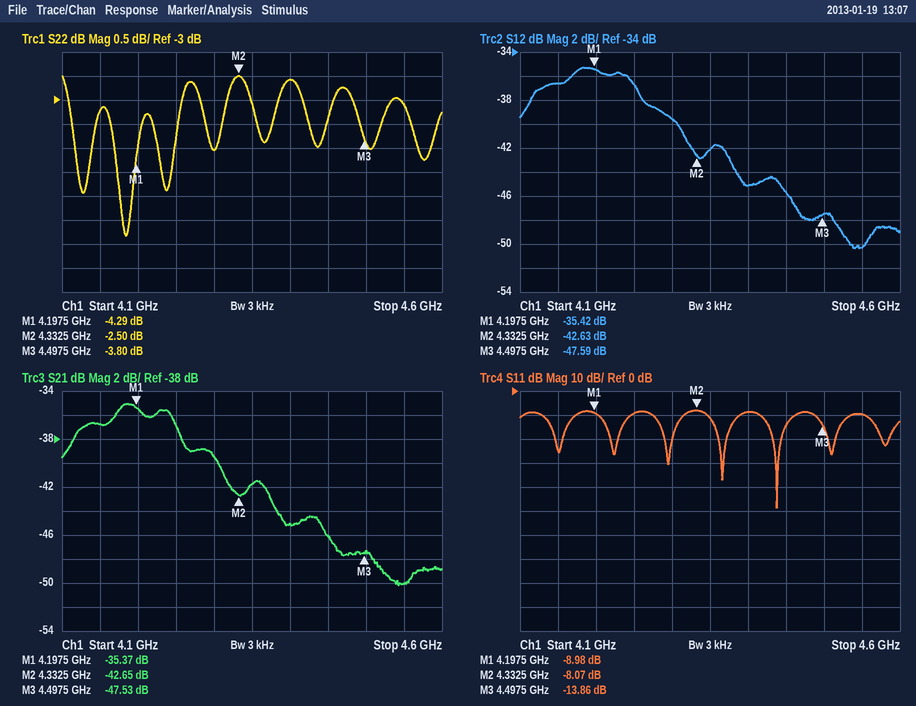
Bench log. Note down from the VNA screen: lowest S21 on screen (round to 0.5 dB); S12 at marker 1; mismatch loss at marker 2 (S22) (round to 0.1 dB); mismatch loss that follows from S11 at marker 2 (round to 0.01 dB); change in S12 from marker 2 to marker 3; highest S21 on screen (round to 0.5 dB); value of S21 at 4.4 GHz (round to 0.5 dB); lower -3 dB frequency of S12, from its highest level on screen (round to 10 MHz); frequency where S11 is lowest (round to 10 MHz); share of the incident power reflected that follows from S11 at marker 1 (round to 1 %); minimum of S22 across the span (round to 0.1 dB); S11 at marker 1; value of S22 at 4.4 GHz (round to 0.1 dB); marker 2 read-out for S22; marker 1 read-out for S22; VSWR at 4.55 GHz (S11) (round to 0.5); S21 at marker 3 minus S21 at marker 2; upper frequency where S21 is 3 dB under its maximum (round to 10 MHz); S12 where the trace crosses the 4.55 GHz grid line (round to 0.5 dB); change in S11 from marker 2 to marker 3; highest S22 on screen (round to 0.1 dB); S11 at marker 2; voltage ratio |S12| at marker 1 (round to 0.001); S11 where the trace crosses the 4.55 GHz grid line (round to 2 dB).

-50.0 dB
-35.42 dB
3.6 dB
0.74 dB
-4.96 dB
-35.0 dB
-45.0 dB
4.11 GHz
4.44 GHz
13 %
-5.8 dB
-8.98 dB
-2.6 dB
-2.50 dB
-4.29 dB
2.0
-4.88 dB
4.26 GHz
-50.5 dB
-5.79 dB
-2.5 dB
-8.07 dB
0.017
-10 dB
